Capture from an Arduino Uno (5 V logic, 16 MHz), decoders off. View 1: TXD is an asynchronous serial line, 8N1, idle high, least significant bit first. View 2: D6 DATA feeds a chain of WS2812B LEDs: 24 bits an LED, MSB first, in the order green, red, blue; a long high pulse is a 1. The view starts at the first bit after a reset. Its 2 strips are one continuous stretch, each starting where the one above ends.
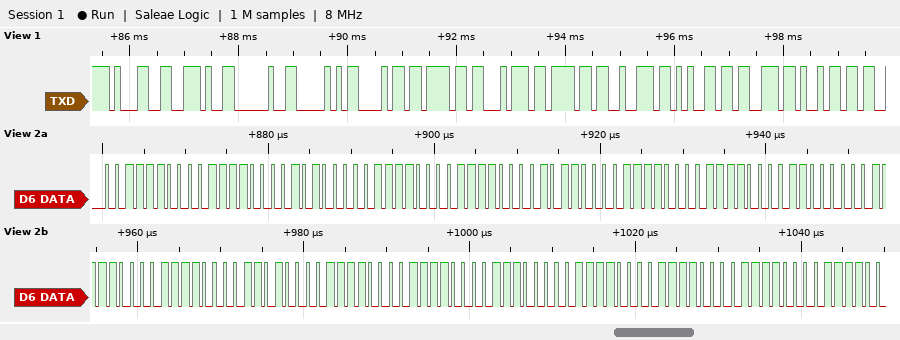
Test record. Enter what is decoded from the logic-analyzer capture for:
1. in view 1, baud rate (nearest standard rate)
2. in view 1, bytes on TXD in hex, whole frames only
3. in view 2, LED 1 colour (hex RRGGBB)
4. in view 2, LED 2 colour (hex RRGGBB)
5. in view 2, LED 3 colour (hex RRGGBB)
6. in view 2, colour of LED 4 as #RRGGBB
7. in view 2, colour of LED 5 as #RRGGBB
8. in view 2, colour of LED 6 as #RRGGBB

9600 baud
31 2E 20 50 68 6F 74 6F 72 65 73 69
#3C3C28
#3C3C2C
#3C3C30
#3C3C34
#3C3C38
#3C3C3C
